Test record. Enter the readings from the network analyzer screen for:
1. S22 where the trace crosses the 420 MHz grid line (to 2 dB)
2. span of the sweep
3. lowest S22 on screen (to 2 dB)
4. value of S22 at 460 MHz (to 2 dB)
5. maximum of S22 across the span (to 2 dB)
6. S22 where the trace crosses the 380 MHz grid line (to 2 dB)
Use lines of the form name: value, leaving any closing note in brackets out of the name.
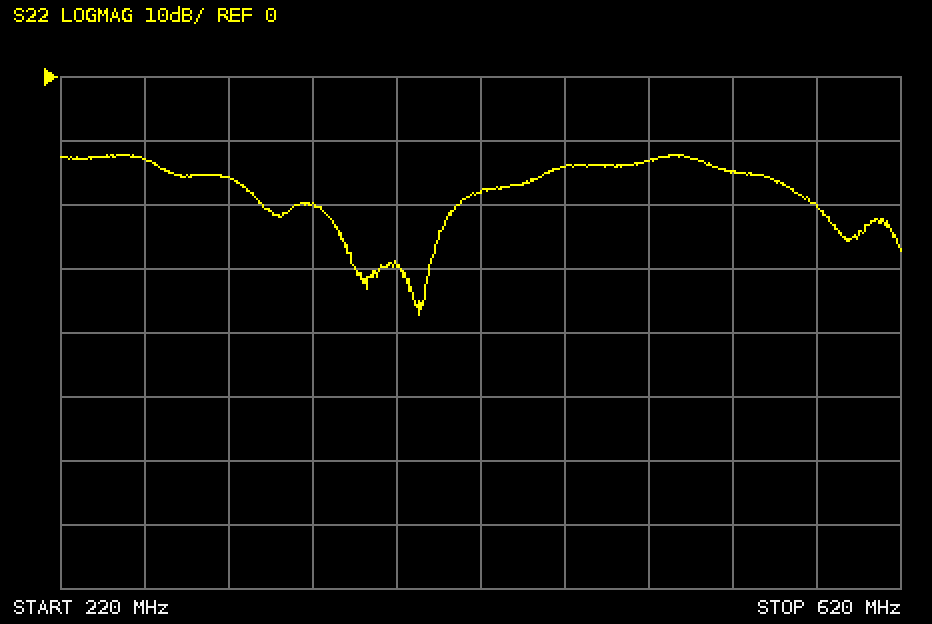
S22 where the trace crosses the 420 MHz grid line: -18 dB
span of the sweep: 400 MHz
lowest S22 on screen: -38 dB
value of S22 at 460 MHz: -14 dB
maximum of S22 across the span: -12 dB
S22 where the trace crosses the 380 MHz grid line: -30 dB
